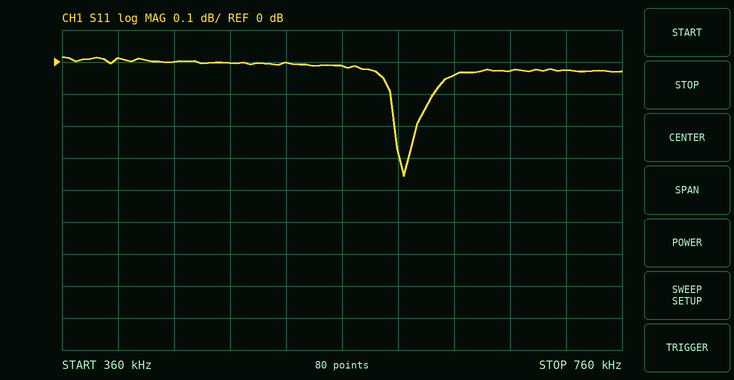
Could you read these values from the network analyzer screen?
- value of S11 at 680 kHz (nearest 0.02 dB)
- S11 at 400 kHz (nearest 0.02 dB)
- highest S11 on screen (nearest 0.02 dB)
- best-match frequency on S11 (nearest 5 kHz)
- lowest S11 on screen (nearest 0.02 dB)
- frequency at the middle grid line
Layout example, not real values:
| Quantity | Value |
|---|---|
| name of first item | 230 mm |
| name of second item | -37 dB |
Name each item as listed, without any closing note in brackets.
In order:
| Quantity | Value |
|---|---|
| value of S11 at 680 kHz | -0.02 dB |
| S11 at 400 kHz | 0.02 dB |
| highest S11 on screen | 0.02 dB |
| best-match frequency on S11 | 605 kHz |
| lowest S11 on screen | -0.36 dB |
| frequency at the middle grid line | 560 kHz |
